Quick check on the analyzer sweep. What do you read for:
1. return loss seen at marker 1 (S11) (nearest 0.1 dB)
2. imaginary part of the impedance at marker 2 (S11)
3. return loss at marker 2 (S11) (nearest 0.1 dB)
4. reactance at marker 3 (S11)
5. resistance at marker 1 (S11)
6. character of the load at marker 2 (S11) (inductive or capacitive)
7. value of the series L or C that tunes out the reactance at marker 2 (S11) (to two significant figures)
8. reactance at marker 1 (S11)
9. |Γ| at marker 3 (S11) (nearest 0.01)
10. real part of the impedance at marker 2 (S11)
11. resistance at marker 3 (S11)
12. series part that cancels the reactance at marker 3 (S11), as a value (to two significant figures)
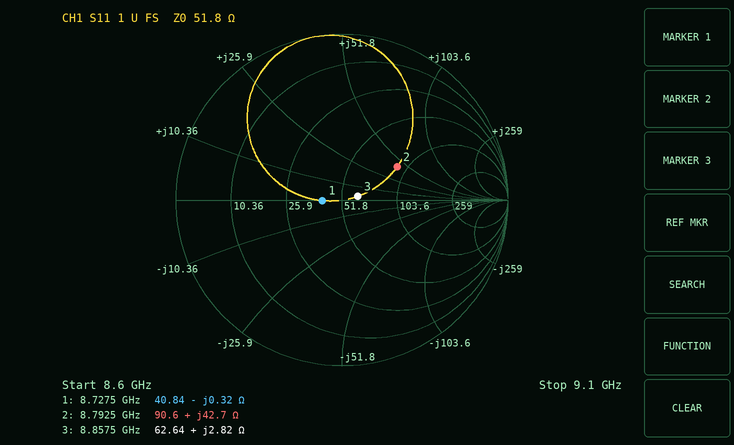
18.5 dB
+42.7 Ω
8.2 dB
+2.82 Ω
40.84 Ω
inductive
420 fF
-0.32 Ω
0.10
90.6 Ω
62.64 Ω
6.4 pF
